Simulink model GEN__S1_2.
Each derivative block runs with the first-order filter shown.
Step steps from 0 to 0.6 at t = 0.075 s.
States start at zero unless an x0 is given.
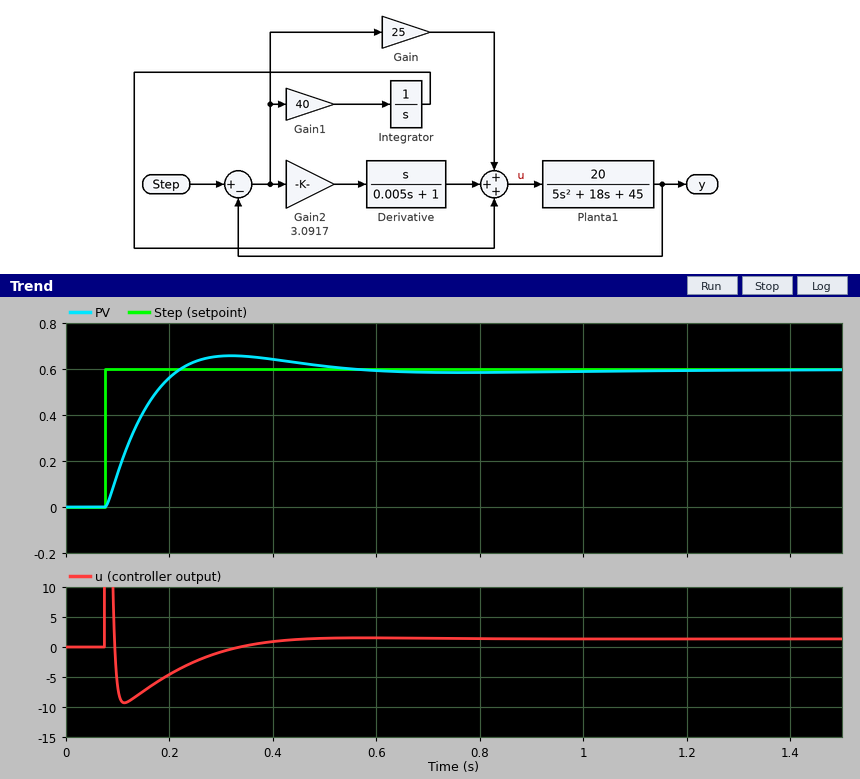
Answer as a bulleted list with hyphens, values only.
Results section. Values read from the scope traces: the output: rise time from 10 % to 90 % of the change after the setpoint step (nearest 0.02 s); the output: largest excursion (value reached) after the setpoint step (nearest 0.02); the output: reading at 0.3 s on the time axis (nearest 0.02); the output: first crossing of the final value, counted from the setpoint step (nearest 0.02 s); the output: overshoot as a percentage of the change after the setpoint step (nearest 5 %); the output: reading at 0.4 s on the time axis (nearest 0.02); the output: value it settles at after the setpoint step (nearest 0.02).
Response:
- 0.10 s
- 0.66
- 0.66
- 0.14 s
- 10 %
- 0.64
- 0.60
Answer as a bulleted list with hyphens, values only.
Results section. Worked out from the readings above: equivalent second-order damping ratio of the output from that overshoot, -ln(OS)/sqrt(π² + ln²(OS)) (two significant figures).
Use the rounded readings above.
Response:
- 0.59
